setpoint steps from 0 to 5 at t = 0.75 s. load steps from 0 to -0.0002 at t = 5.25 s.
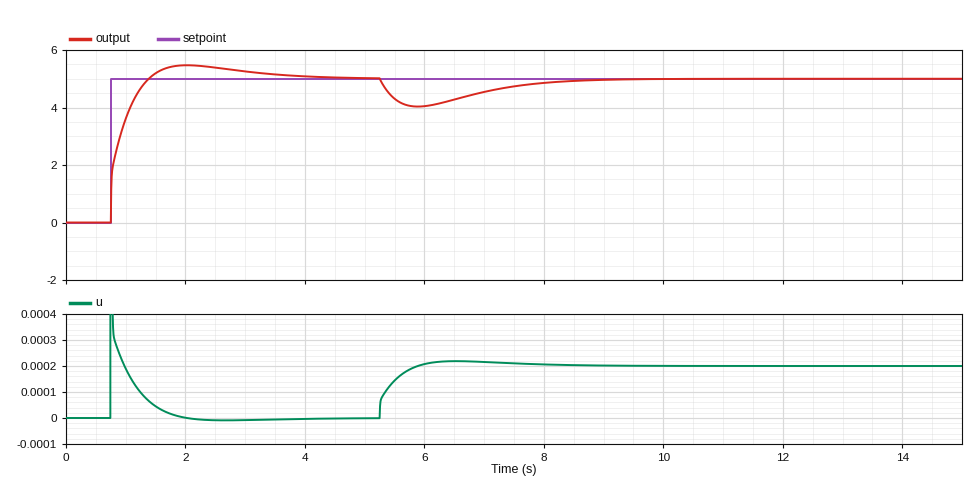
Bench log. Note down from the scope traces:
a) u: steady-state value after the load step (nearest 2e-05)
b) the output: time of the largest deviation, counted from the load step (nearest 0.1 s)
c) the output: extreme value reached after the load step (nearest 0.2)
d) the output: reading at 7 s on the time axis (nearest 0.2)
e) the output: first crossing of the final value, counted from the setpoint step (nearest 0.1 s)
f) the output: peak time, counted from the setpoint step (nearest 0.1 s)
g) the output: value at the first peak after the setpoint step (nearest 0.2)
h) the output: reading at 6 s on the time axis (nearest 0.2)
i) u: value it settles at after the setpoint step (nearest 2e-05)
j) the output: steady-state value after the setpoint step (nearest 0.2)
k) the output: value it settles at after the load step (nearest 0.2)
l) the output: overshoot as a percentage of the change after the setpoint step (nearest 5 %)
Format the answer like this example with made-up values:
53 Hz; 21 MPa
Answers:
0.00020; 0.6 s; 4.0; 4.6; 0.6 s; 1.3 s; 5.4; 4.0; 0.00000; 5.0; 5.0; 10 %
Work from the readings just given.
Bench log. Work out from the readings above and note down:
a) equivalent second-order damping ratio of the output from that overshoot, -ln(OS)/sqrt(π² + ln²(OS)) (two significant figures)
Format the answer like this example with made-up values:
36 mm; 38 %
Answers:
0.59
